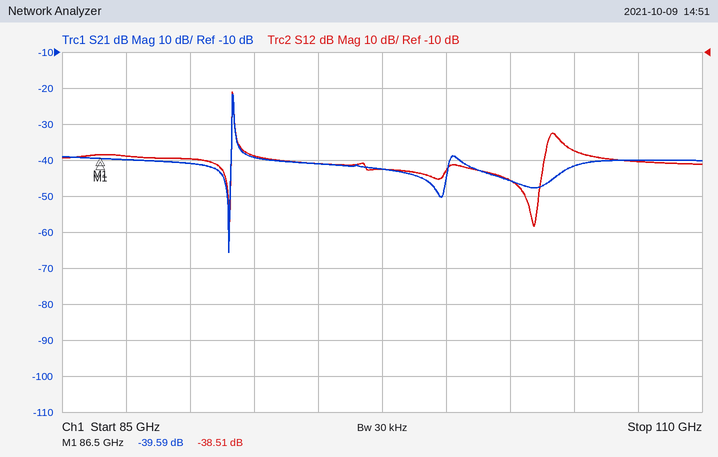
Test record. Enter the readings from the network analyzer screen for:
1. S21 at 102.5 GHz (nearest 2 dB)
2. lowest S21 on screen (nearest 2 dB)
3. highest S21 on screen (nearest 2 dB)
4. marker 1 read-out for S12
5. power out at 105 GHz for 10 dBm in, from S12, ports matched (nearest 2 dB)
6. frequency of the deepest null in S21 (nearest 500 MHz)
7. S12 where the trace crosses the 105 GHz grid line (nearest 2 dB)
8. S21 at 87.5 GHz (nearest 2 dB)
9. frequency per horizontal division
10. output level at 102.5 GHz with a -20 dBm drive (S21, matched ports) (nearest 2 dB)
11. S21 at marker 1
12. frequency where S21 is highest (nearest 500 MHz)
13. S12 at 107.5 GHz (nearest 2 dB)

-46 dB
-66 dB
-22 dB
-38.51 dB
-28 dBm
91.5 GHz
-38 dB
-40 dB
2.5 GHz
-66 dBm
-39.59 dB
91.5 GHz
-40 dB
